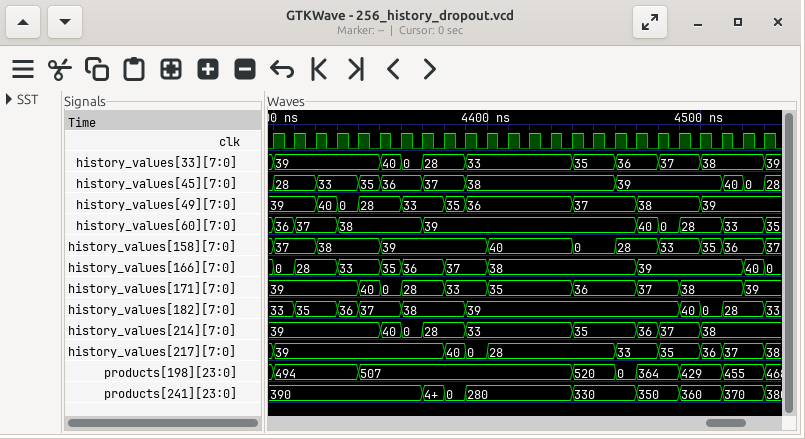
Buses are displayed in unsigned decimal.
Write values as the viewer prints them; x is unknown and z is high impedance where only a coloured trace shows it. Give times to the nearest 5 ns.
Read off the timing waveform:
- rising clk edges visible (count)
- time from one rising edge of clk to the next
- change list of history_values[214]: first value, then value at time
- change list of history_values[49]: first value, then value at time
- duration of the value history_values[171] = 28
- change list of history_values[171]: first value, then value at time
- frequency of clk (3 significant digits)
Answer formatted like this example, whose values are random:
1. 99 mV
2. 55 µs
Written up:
1. 24
2. 10 ns
3. 39, 40 at 4350 ns, 0 at 4360 ns, 28 at 4370 ns, 33 at 4390 ns, 35 at 4440 ns, 36 at 4470 ns, 37 at 4480 ns, 38 at 4500 ns
4. 39, 40 at 4320 ns, 0 at 4330 ns, 28 at 4340 ns, 33 at 4360 ns, 35 at 4380 ns, 36 at 4390 ns, 37 at 4440 ns, 38 at 4470 ns, 39 at 4500 ns
5. 20 ns
6. 39, 40 at 4340 ns, 0 at 4350 ns, 28 at 4360 ns, 33 at 4380 ns, 35 at 4400 ns, 36 at 4440 ns, 37 at 4470 ns, 38 at 4490 ns, 39 at 4520 ns
7. 100 MHz
